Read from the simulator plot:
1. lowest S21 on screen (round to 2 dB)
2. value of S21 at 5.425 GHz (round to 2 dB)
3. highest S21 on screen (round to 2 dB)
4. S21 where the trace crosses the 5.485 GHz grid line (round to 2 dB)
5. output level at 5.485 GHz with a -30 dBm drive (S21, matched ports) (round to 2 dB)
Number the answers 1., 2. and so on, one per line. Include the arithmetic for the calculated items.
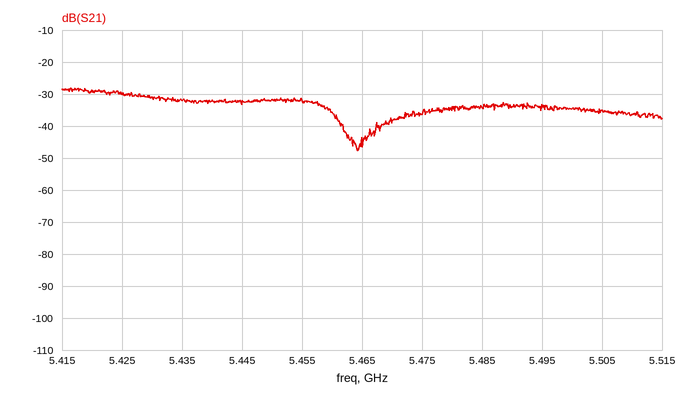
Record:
1. -48 dB
2. -30 dB
3. -28 dB
4. -34 dB
5. -30 dBm + (-34 dB) = -64 dBm
